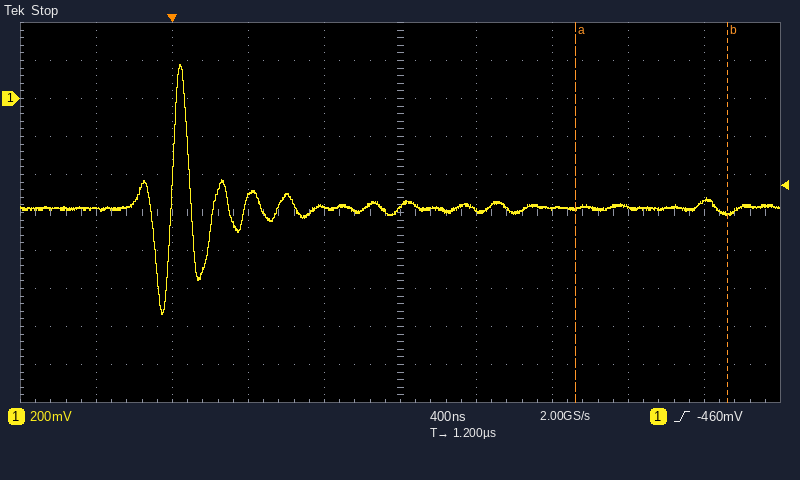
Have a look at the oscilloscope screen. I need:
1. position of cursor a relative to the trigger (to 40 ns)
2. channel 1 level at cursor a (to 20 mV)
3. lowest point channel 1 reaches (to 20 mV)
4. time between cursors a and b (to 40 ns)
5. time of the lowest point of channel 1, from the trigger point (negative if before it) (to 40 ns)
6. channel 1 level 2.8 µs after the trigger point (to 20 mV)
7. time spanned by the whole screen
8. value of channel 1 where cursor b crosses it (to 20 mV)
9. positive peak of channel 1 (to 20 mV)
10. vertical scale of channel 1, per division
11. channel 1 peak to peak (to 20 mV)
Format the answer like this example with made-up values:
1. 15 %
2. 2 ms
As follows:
1. +2.12 µs
2. -580 mV
3. -1.14 V
4. 800 ns
5. -40 ns
6. -540 mV
7. 4 µs
8. -600 mV
9. 180 mV
10. 200 mV
11. 1.32 V
